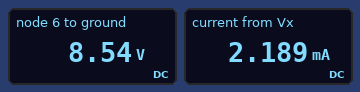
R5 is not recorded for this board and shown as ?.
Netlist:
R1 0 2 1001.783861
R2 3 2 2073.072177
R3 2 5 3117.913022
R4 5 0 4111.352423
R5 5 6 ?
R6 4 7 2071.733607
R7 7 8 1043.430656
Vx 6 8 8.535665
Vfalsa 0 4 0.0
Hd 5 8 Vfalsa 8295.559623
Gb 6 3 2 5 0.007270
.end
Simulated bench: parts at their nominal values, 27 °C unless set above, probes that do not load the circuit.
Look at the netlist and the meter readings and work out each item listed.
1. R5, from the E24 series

3.9 kΩ
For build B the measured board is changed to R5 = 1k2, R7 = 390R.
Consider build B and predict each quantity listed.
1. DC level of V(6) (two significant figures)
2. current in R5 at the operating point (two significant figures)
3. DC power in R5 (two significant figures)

8.5 V
7.1 mA
61 mW
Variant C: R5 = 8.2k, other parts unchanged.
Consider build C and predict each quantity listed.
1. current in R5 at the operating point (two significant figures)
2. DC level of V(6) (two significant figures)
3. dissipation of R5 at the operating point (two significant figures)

1.0 mA
8.5 V
8.9 mW
